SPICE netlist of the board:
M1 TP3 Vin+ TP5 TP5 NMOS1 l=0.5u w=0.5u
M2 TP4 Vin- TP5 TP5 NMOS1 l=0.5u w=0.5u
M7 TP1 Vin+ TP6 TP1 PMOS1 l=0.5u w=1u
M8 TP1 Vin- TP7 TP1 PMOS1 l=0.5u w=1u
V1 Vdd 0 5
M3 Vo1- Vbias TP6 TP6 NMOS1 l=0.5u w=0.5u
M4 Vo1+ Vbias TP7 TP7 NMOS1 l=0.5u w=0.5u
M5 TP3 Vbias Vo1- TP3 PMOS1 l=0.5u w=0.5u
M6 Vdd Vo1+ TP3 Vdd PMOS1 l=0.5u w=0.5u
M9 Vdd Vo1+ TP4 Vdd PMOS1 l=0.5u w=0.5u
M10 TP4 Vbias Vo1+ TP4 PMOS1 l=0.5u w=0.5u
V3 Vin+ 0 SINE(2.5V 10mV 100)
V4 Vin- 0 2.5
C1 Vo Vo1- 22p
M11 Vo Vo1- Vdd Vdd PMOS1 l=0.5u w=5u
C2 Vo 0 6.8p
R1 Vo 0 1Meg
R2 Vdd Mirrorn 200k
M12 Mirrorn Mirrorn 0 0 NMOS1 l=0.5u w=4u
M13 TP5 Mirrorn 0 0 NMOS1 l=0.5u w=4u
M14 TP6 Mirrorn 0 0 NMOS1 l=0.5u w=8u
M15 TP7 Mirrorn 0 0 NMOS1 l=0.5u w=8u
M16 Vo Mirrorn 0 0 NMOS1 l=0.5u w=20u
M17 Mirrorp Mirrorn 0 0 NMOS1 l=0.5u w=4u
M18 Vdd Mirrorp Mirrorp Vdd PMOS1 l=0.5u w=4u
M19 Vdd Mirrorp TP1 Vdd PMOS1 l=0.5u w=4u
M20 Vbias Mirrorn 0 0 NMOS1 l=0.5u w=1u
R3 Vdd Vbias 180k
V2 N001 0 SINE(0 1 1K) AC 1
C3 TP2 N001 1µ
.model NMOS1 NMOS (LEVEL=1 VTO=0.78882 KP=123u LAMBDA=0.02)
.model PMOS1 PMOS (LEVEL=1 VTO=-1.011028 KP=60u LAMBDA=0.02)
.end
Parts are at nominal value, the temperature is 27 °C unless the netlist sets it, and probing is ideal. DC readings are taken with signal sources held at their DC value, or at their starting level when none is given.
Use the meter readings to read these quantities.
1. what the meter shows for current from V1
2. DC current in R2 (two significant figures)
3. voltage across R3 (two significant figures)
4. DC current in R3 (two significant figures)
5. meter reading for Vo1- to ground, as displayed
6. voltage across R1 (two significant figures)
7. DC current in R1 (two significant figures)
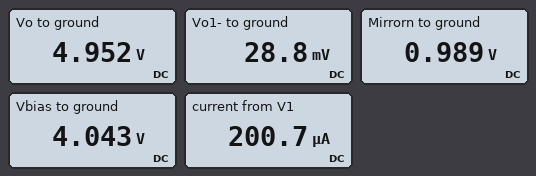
200.7 µA
20 µA
960 mV
5.3 µA
28.8 mV
5.0 V
5.0 µA
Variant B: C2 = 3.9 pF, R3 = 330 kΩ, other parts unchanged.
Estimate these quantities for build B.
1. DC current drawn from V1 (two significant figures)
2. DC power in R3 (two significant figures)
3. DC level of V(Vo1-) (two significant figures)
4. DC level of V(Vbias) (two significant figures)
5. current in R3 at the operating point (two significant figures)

230 µA
9.1 µW
110 mV
3.3 V
5.2 µA
